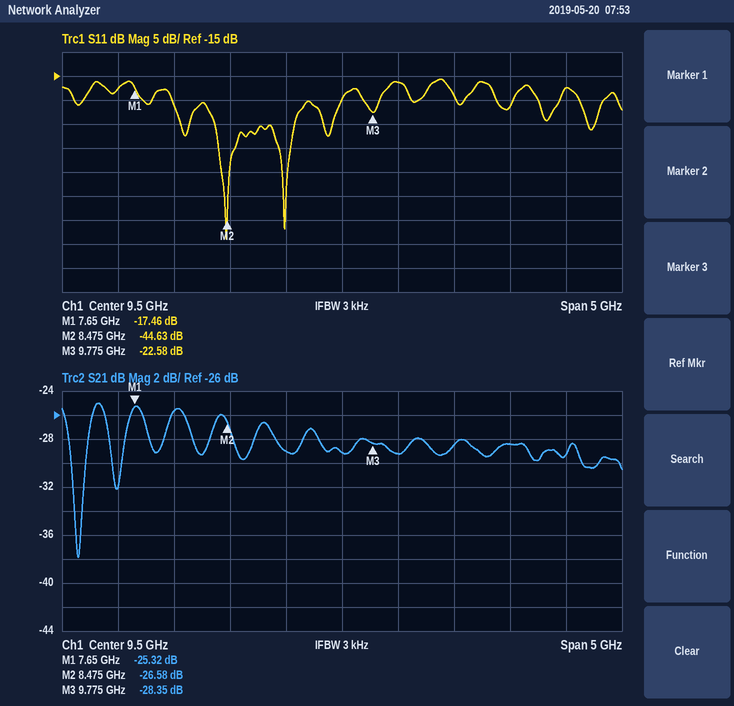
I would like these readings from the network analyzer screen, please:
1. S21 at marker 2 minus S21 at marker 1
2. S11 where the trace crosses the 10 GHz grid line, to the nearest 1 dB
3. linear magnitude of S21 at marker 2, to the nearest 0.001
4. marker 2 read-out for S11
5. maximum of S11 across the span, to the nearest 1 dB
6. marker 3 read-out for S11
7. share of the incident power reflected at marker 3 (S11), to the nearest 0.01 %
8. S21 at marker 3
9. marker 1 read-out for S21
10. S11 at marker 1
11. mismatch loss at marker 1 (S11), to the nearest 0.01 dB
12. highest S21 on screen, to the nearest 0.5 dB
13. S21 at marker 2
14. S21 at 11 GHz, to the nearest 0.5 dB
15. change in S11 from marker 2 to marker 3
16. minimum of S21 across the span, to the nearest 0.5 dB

-1.26 dB
-16 dB
0.047
-44.63 dB
-16 dB
-22.58 dB
0.55 %
-28.35 dB
-25.32 dB
-17.46 dB
0.08 dB
-25.0 dB
-26.58 dB
-28.5 dB
22.05 dB
-38.0 dB
